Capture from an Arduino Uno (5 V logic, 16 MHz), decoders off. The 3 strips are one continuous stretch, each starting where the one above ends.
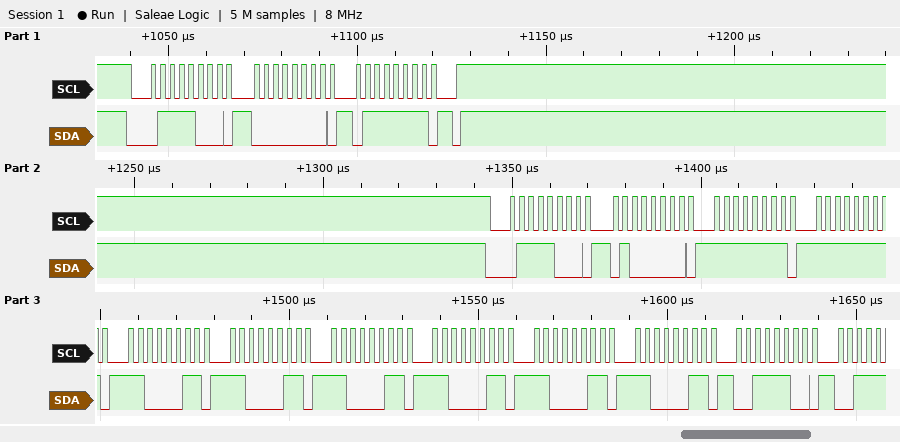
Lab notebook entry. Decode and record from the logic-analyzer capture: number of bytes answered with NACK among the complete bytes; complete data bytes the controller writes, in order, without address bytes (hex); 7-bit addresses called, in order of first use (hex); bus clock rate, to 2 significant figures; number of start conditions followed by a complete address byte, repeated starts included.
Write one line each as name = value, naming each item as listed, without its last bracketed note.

number of bytes answered with NACK among the complete bytes = 0
complete data bytes the controller writes, in order, without address bytes = 00 7F 40 FF FF C3 C3 C3 C3 C3 C3 3C
7-bit addresses called, in order of first use = 0x3C
bus clock rate, to 2 significant figures = 400 kHz
number of start conditions followed by a complete address byte, repeated starts included = 2
